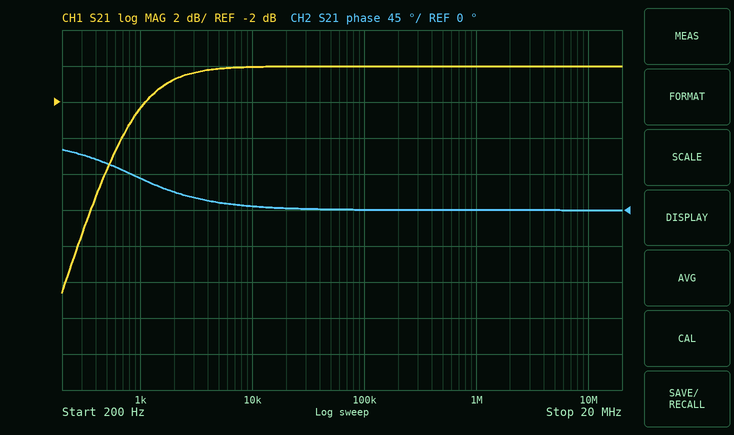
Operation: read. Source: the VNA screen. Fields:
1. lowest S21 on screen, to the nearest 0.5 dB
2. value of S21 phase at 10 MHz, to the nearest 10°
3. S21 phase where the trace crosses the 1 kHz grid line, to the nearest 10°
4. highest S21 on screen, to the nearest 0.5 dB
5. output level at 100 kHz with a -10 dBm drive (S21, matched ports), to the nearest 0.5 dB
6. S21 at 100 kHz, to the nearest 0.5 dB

-12.5 dB
0°
40°
0.0 dB
-10.0 dBm
0.0 dB
